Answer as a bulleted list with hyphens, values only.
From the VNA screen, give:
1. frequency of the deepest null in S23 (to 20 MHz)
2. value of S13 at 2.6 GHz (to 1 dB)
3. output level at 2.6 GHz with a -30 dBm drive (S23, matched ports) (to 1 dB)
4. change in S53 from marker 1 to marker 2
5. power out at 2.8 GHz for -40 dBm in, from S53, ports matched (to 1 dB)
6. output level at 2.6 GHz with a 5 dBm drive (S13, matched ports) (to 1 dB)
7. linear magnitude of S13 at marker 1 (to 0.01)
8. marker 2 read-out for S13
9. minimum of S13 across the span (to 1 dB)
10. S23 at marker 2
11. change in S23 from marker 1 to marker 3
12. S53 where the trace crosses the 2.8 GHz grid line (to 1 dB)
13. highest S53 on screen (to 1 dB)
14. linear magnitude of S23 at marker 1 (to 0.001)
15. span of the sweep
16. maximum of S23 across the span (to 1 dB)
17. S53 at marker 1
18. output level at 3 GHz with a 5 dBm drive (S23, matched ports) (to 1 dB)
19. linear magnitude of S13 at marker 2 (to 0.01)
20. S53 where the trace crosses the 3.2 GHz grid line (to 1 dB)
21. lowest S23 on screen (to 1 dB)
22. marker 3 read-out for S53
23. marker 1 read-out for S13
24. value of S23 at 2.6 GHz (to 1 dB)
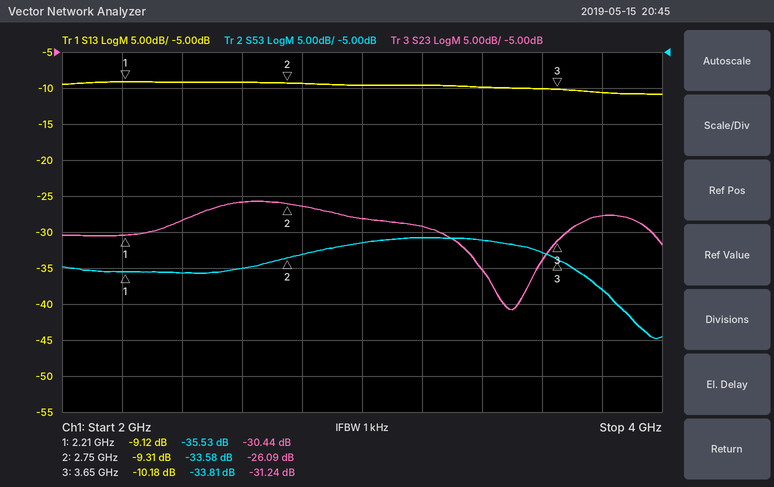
- 3.50 GHz
- -9 dB
- -56 dBm
- 1.95 dB
- -73 dBm
- -4 dBm
- 0.35
- -9.31 dB
- -11 dB
- -26.09 dB
- -0.80 dB
- -33 dB
- -31 dB
- 0.030
- 2 GHz
- -26 dB
- -35.53 dB
- -23 dBm
- 0.34
- -31 dB
- -41 dB
- -33.81 dB
- -9.12 dB
- -26 dB
